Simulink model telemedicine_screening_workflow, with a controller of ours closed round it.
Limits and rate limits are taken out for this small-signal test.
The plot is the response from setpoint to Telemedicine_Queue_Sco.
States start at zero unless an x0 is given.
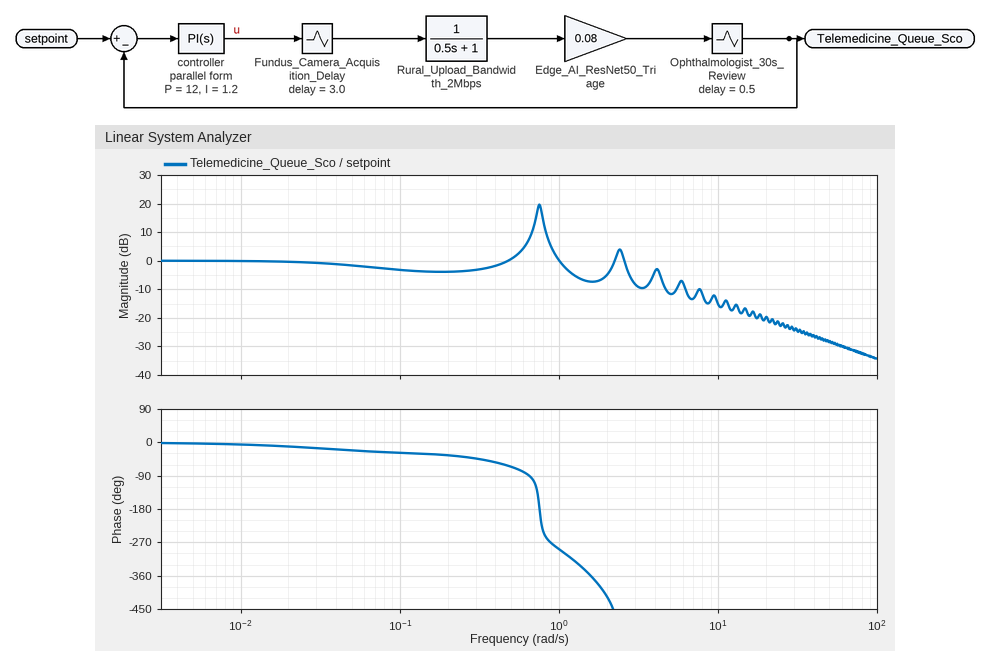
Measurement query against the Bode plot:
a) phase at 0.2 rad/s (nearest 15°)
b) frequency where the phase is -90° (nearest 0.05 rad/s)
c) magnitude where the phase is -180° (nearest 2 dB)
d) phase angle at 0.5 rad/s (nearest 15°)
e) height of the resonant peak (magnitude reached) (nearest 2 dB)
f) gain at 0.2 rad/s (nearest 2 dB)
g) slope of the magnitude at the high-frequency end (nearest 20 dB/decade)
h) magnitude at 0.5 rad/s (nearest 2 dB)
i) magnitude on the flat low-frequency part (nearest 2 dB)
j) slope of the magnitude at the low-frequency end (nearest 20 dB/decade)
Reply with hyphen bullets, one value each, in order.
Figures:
- -30°
- 0.65 rad/s
- 20 dB
- -60°
- 20 dB
- -4 dB
- -20 dB/decade
- 0 dB
- 0 dB
- 0 dB/decade
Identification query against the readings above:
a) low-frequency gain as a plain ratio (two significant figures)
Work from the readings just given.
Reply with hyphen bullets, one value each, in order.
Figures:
- 1.0
